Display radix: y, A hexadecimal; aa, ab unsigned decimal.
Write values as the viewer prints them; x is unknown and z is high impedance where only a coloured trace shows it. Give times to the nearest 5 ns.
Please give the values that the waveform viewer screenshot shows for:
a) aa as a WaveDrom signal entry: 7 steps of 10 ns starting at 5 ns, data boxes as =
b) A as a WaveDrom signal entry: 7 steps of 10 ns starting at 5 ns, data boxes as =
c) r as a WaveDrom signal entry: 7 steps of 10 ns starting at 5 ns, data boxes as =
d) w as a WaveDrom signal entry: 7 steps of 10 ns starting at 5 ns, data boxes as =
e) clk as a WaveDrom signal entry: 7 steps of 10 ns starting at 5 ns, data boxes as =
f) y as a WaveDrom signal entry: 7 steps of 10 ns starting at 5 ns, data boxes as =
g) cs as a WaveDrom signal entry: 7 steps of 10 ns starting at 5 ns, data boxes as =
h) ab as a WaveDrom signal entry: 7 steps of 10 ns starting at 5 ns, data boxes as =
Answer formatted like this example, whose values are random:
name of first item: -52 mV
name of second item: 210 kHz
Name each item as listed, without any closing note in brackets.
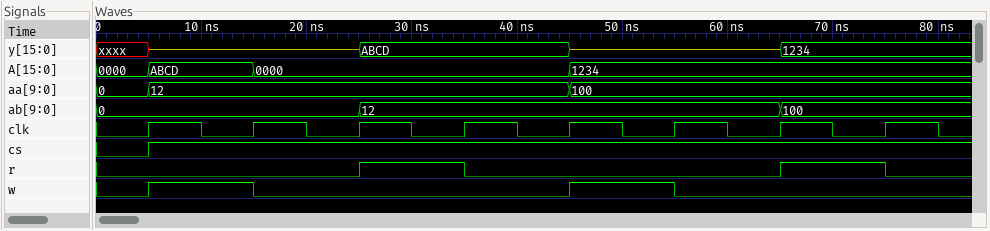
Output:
aa as a WaveDrom signal entry: 7 steps of 10 ns starting at 5 ns, data boxes as =: {name: 'aa', wave: '=...=..', data: '12 100'}
A as a WaveDrom signal entry: 7 steps of 10 ns starting at 5 ns, data boxes as =: {name: 'A', wave: '==..=..', data: 'ABCD 0000 1234'}
r as a WaveDrom signal entry: 7 steps of 10 ns starting at 5 ns, data boxes as =: {name: 'r', wave: '0.10..1'}
w as a WaveDrom signal entry: 7 steps of 10 ns starting at 5 ns, data boxes as =: {name: 'w', wave: '10..10.'}
clk as a WaveDrom signal entry: 7 steps of 10 ns starting at 5 ns, data boxes as =: {name: 'clk', wave: 'p......'}
y as a WaveDrom signal entry: 7 steps of 10 ns starting at 5 ns, data boxes as =: {name: 'y', wave: 'z.=.z.=', data: 'ABCD 1234'}
cs as a WaveDrom signal entry: 7 steps of 10 ns starting at 5 ns, data boxes as =: {name: 'cs', wave: '1......'}
ab as a WaveDrom signal entry: 7 steps of 10 ns starting at 5 ns, data boxes as =: {name: 'ab', wave: '=.=...=', data: '0 12 100'}
